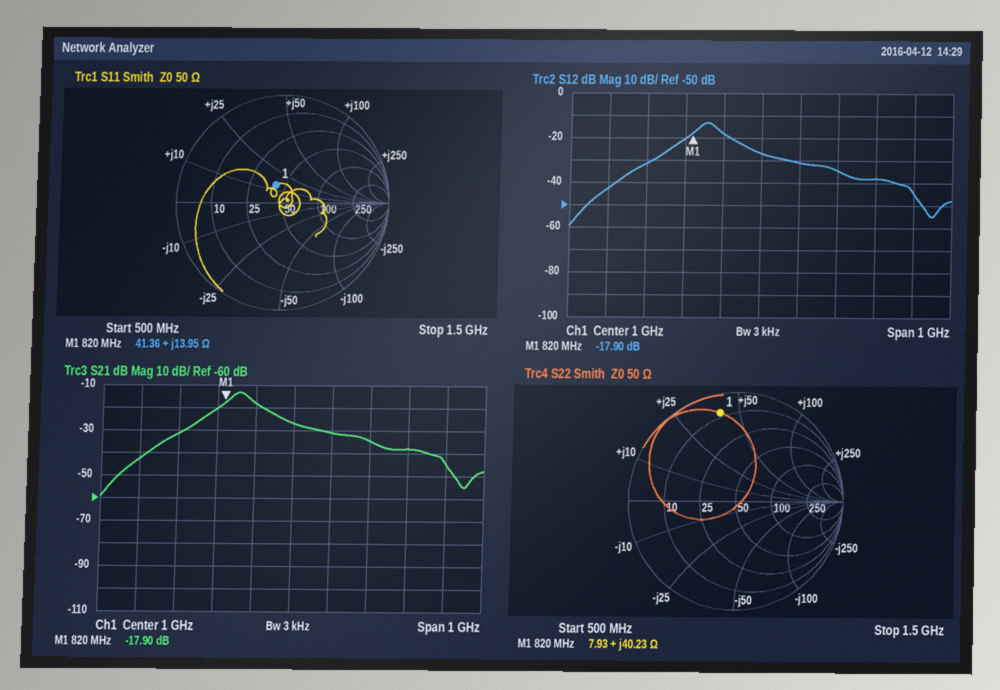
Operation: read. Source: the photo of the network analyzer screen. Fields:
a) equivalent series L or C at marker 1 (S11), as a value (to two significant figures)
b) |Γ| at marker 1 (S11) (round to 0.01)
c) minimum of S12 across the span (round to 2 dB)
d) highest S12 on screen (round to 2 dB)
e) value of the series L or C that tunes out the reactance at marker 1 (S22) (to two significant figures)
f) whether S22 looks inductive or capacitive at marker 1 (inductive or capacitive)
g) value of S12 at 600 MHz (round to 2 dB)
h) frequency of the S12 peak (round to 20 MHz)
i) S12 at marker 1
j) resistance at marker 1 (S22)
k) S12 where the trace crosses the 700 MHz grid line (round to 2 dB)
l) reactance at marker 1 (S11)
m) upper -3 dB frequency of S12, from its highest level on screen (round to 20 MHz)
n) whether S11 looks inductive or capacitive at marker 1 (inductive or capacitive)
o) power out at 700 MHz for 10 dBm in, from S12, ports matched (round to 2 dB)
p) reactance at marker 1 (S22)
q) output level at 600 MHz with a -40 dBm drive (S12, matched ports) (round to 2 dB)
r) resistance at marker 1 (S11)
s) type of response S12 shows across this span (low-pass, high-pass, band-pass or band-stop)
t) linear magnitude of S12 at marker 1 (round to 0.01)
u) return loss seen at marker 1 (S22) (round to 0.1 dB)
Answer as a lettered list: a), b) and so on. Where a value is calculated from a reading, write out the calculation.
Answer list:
a) L = 13.95 Ω/(2π × 820 MHz) ≈ 2.7 nH
b) 0.18
c) -60 dB
d) -14 dB
e) C = 1/(2π × 820 MHz × 40.23 Ω) ≈ 4.8 pF
f) inductive
g) -42 dB
h) 860 MHz
i) -17.90 dB
j) 7.93 Ω
k) -32 dB
l) +13.95 Ω
m) 880 MHz
n) inductive
o) 10 dBm + (-32 dB) = -22 dBm
p) +40.23 Ω
q) -40 dBm + (-42 dB) = -82 dBm
r) 41.36 Ω
s) band-pass
t) 10^(-17.9/20) ≈ 0.13
u) 1.7 dB
